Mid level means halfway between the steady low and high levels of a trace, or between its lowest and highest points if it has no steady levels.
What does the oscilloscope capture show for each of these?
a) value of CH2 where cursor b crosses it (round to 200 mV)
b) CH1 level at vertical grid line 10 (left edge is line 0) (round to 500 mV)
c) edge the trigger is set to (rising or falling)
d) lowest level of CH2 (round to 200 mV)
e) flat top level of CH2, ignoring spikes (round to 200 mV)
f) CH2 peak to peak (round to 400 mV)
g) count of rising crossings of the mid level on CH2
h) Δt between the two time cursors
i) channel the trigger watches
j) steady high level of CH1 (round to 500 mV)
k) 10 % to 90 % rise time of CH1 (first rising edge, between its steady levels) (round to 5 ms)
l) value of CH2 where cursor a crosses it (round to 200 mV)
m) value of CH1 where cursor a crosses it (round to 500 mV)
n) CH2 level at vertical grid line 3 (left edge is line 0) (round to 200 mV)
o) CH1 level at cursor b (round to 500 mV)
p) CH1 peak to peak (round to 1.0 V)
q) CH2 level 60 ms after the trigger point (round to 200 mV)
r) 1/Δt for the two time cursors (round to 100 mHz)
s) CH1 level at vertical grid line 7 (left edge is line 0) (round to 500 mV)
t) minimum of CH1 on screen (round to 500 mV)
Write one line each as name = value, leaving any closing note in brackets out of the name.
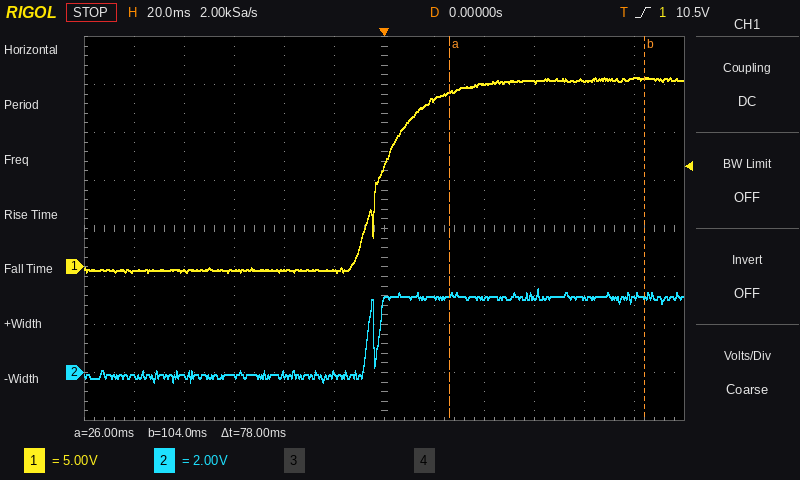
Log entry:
value of CH2 where cursor b crosses it = 3.2 V
CH1 level at vertical grid line 10 (left edge is line 0) = 19.5 V
edge the trigger is set to = rising
lowest level of CH2 = -400 mV
flat top level of CH2, ignoring spikes = 3.2 V
CH2 peak to peak = 4.0 V
count of rising crossings of the mid level on CH2 = 2
Δt between the two time cursors = 78 ms
channel the trigger watches = CH1
steady high level of CH1 = 19.5 V
10 % to 90 % rise time of CH1 (first rising edge, between its steady levels) = 30 ms
value of CH2 where cursor a crosses it = 3.2 V
value of CH1 where cursor a crosses it = 18.0 V
CH2 level at vertical grid line 3 (left edge is line 0) = -200 mV
CH1 level at cursor b = 19.5 V
CH1 peak to peak = 20.0 V
CH2 level 60 ms after the trigger point = 3.2 V
1/Δt for the two time cursors = 12.8 Hz
CH1 level at vertical grid line 7 (left edge is line 0) = 17.5 V
minimum of CH1 on screen = -500 mV
